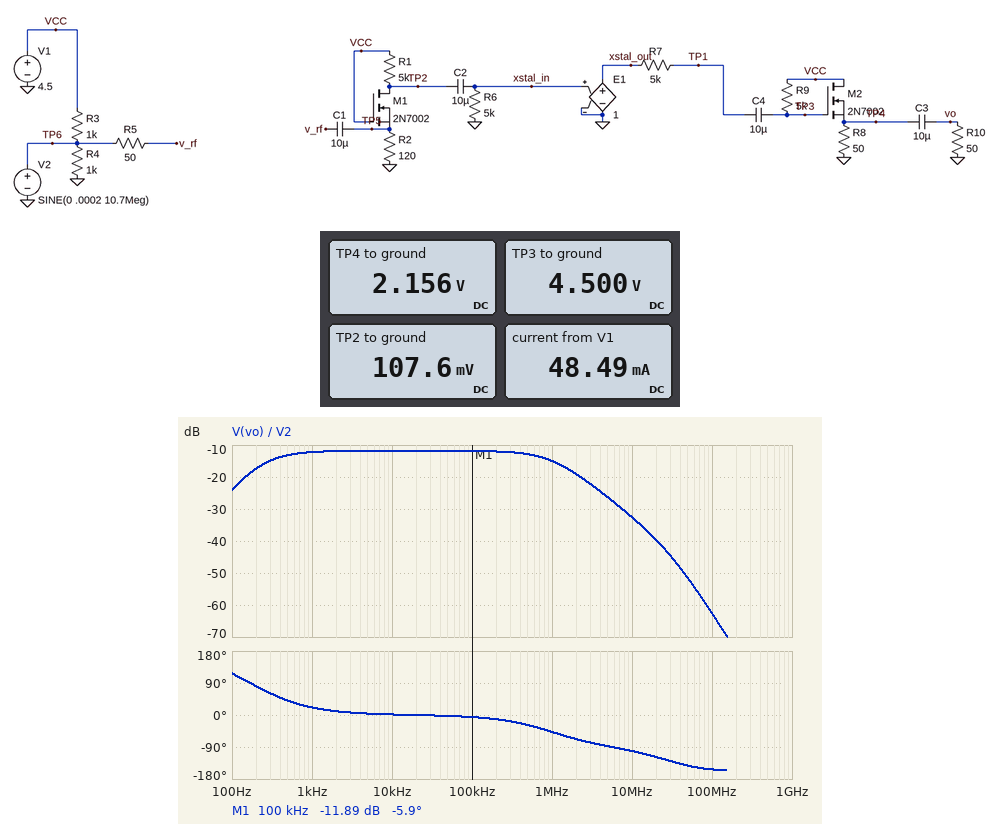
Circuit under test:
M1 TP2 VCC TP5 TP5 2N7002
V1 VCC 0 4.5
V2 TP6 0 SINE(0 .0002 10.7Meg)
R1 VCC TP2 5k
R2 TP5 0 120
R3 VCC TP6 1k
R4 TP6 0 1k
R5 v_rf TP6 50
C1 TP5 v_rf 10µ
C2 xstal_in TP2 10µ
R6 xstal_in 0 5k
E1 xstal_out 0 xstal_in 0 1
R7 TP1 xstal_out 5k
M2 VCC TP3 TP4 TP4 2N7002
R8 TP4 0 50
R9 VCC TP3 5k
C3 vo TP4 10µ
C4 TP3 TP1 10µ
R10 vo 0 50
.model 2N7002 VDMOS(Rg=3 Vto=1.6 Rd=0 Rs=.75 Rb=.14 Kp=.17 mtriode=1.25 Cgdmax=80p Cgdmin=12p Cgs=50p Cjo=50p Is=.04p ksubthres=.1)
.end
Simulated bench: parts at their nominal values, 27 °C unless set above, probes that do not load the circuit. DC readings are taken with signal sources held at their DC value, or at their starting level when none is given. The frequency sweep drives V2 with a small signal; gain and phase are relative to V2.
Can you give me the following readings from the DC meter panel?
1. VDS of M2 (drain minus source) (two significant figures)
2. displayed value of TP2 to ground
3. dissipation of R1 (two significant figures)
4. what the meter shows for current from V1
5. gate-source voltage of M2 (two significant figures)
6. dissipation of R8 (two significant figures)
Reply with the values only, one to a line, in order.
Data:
2.3 V
107.6 mV
3.9 mW
48.49 mA
2.3 V
93 mW
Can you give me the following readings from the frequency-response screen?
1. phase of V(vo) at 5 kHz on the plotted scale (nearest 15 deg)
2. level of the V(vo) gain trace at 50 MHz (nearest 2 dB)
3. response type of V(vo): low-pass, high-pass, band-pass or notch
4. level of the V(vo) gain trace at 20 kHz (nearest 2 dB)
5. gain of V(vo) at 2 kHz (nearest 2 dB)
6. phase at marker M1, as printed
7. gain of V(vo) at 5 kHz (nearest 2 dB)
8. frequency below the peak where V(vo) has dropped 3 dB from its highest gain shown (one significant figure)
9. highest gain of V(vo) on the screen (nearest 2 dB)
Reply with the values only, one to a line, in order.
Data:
0 deg
-52 dB
band-pass
-12 dB
-12 dB
-5.9 deg
-12 dB
300 Hz
-12 dB
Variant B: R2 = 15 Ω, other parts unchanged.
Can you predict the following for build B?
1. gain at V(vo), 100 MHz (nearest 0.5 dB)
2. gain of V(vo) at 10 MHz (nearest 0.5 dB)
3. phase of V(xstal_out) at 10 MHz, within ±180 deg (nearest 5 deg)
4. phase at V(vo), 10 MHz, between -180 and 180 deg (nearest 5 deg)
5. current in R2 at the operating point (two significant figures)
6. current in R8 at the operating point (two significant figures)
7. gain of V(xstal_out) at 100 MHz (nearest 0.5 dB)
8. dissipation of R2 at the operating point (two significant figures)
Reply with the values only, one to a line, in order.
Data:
-66.0 dB
-42.0 dB
-5 deg
-90 deg
900 µA
43 mA
-17.0 dB
12 µW
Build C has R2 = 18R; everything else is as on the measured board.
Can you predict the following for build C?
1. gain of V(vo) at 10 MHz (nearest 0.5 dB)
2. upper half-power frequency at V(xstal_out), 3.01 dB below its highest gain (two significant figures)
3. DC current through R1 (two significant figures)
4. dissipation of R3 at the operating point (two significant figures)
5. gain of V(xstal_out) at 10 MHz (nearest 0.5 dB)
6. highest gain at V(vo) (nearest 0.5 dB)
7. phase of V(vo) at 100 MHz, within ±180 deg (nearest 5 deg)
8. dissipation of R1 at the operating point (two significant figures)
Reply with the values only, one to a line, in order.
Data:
-40.5 dB
71 MHz
900 µA
20 mW
-11.5 dB
-20.5 dB
-135 deg
4.0 mW
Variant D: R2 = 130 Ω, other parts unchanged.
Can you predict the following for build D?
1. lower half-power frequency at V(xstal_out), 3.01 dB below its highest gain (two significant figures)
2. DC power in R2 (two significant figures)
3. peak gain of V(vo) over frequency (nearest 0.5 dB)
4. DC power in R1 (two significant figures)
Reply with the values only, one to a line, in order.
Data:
92 Hz
100 µW
-11.5 dB
3.8 mW
